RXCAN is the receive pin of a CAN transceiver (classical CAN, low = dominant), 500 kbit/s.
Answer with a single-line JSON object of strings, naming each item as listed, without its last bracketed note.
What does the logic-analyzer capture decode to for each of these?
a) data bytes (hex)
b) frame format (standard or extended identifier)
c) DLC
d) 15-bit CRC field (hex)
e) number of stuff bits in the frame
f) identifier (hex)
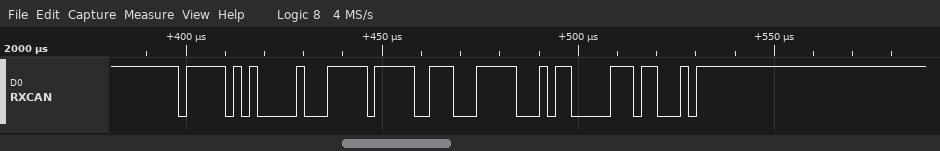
{"data bytes": "FF 71 F2", "frame format": "standard", "DLC": "3", "15-bit CRC field": "0x60D8", "number of stuff bits in the frame": "6", "identifier": "0x7E8"}
